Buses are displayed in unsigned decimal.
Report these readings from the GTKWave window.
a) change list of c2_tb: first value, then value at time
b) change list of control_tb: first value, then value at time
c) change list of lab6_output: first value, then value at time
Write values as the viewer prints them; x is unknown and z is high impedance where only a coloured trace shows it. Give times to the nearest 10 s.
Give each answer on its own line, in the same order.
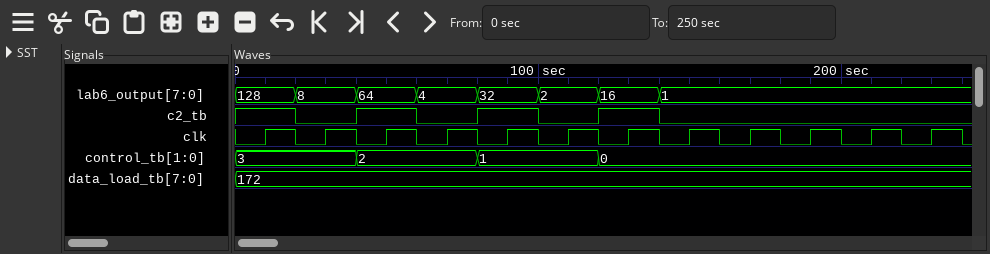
1, 0 at 20 s, 1 at 40 s, 0 at 60 s, 1 at 80 s, 0 at 100 s, 1 at 120 s, 0 at 140 s
3, 2 at 40 s, 1 at 80 s, 0 at 120 s
128, 8 at 20 s, 64 at 40 s, 4 at 60 s, 32 at 80 s, 2 at 100 s, 16 at 120 s, 1 at 140 s
